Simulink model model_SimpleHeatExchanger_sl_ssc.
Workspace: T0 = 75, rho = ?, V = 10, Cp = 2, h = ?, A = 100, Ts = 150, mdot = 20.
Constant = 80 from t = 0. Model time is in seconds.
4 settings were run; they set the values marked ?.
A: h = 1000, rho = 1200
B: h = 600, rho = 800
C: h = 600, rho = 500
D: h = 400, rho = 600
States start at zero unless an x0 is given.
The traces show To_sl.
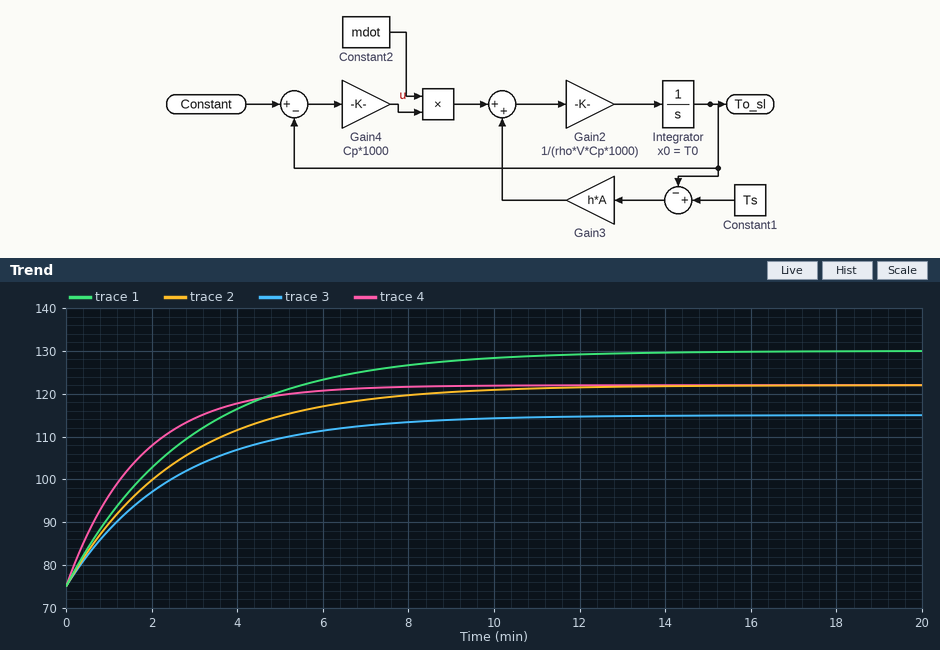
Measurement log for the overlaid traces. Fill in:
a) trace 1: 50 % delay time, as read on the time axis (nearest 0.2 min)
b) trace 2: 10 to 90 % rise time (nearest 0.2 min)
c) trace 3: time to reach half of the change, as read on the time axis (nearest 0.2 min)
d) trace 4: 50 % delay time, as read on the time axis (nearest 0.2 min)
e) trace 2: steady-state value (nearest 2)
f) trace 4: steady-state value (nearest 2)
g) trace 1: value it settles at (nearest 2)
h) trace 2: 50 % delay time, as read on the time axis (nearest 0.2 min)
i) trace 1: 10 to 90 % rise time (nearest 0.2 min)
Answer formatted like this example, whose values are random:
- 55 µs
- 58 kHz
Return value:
- 2.0 min
- 5.8 min
- 1.8 min
- 1.2 min
- 122
- 122
- 130
- 1.8 min
- 6.2 min
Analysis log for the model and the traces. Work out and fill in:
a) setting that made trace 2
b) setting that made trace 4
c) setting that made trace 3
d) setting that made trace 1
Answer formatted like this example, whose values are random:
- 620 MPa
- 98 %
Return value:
- B
- C
- D
- A
